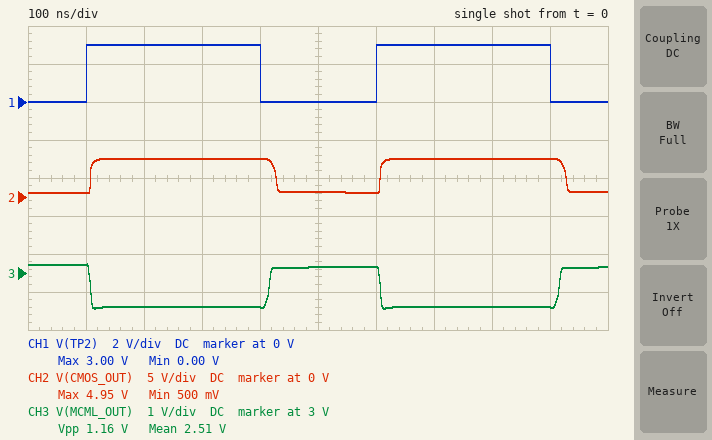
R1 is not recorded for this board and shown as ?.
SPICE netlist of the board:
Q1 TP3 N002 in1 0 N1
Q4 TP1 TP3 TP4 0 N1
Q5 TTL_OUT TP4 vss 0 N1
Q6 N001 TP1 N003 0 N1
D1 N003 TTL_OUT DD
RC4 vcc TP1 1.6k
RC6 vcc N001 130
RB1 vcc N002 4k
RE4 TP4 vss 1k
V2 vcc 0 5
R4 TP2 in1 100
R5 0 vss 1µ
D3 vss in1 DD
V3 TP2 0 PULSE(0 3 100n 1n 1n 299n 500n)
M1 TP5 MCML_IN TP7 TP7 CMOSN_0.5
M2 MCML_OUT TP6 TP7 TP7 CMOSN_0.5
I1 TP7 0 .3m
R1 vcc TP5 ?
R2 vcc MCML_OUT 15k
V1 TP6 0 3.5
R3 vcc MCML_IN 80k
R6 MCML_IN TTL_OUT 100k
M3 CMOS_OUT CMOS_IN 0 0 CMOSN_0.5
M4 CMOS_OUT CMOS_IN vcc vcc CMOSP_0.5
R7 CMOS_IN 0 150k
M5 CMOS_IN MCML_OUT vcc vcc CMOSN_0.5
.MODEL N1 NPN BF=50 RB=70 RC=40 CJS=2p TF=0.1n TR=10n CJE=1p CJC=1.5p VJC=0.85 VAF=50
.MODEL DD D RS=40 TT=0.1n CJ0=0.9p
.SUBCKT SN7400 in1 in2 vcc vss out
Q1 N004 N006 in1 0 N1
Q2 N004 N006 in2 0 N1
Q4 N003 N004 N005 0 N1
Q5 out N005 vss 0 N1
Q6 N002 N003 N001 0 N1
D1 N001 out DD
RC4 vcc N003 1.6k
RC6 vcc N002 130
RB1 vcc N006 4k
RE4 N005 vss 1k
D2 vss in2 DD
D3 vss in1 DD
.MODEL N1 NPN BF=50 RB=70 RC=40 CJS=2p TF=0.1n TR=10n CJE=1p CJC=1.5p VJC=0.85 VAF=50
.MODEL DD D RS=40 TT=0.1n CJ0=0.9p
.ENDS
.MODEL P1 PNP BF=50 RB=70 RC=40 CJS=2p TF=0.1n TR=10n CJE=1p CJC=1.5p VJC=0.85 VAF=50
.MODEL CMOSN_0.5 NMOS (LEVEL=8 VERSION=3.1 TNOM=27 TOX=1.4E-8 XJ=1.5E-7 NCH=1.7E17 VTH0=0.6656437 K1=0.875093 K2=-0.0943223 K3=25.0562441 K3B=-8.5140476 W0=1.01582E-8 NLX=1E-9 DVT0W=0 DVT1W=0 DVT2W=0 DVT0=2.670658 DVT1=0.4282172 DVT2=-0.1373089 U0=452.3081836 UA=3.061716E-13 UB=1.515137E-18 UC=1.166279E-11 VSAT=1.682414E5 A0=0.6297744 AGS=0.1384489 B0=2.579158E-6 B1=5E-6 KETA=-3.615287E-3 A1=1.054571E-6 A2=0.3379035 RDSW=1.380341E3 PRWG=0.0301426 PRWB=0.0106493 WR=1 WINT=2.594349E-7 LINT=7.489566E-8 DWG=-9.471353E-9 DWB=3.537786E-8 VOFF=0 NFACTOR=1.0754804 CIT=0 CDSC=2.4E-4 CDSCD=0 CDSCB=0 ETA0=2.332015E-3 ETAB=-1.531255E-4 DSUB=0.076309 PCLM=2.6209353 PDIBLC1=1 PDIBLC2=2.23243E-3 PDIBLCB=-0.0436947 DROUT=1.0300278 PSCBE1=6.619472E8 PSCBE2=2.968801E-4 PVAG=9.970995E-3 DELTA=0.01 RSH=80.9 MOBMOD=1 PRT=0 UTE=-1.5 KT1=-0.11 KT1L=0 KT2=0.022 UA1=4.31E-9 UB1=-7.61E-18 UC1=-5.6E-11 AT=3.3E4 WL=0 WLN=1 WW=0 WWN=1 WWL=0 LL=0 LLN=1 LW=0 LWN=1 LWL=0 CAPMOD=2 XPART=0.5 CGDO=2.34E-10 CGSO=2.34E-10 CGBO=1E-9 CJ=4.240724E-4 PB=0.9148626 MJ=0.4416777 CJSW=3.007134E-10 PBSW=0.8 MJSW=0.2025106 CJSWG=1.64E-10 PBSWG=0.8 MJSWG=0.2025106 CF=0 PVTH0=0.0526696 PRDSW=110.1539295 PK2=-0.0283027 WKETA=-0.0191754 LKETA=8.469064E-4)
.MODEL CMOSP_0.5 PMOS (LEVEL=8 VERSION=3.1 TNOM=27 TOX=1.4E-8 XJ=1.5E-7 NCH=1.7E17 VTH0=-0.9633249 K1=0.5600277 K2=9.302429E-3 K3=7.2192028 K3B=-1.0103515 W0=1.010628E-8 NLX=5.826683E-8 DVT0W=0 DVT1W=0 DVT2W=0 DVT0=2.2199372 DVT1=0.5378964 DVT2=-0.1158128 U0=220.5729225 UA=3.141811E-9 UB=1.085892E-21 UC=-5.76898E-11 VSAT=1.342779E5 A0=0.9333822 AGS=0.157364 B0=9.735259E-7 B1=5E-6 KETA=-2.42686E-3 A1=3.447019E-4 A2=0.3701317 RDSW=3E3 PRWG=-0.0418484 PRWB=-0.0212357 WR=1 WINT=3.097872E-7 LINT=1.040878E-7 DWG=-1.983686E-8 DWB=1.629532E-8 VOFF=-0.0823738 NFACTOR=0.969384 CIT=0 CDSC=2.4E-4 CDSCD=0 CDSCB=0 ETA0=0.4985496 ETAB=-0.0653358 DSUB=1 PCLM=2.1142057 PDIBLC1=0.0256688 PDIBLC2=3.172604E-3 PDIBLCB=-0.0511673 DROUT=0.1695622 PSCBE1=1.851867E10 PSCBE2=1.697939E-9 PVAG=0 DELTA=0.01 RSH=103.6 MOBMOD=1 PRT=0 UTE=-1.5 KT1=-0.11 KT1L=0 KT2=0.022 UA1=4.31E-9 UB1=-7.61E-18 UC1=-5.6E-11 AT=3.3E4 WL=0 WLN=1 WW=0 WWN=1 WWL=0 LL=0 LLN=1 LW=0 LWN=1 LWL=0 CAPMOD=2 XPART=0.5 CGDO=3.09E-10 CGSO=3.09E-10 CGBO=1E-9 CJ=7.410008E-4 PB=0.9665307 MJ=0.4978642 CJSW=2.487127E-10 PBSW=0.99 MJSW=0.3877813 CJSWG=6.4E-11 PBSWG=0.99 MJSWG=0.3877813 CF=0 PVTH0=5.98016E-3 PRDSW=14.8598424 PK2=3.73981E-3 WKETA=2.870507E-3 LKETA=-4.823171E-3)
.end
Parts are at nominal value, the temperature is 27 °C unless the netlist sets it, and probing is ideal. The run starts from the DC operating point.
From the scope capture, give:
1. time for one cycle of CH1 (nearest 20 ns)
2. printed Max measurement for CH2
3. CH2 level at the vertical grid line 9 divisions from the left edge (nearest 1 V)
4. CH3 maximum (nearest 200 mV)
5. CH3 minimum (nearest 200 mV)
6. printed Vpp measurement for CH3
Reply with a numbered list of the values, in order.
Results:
1. 500 ns
2. 4.95 V
3. 5 V
4. 3.2 V
5. 2.0 V
6. 1.16 V
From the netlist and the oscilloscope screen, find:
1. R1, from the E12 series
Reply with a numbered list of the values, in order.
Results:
1. 18 kΩ
